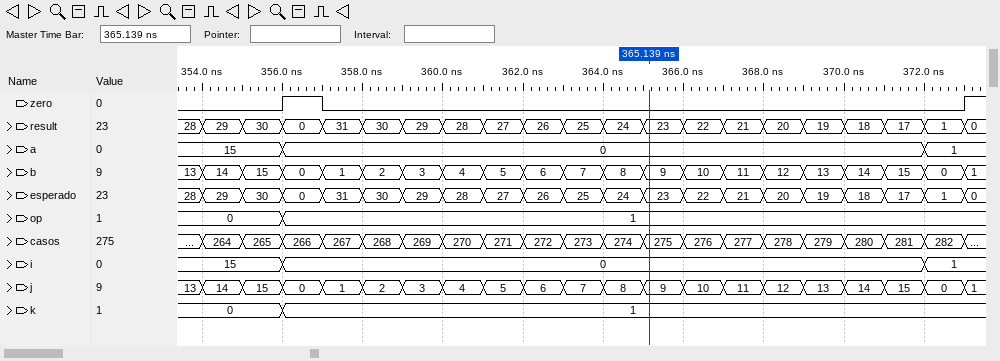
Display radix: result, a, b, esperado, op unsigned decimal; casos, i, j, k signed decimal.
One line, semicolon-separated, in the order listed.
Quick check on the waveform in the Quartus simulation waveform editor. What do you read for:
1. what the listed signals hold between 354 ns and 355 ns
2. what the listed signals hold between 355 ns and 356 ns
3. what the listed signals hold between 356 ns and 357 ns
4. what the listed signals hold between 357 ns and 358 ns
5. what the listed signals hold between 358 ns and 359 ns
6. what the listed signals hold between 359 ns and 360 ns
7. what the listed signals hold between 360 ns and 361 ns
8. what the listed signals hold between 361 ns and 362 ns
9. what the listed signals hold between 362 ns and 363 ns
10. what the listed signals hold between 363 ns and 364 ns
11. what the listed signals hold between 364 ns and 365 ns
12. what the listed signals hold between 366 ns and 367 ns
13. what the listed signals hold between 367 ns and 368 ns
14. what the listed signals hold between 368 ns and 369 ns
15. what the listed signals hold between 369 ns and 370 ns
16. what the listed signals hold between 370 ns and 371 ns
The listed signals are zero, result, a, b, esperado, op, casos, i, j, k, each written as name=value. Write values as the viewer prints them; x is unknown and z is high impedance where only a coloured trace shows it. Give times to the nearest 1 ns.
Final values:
zero=0, result=29, a=15, b=14, esperado=29, op=0, casos=264, i=15, j=14, k=0; zero=0, result=30, a=15, b=15, esperado=30, op=0, casos=265, i=15, j=15, k=0; zero=1, result=0, a=0, b=0, esperado=0, op=1, casos=266, i=0, j=0, k=1; zero=0, result=31, a=0, b=1, esperado=31, op=1, casos=267, i=0, j=1, k=1; zero=0, result=30, a=0, b=2, esperado=30, op=1, casos=268, i=0, j=2, k=1; zero=0, result=29, a=0, b=3, esperado=29, op=1, casos=269, i=0, j=3, k=1; zero=0, result=28, a=0, b=4, esperado=28, op=1, casos=270, i=0, j=4, k=1; zero=0, result=27, a=0, b=5, esperado=27, op=1, casos=271, i=0, j=5, k=1; zero=0, result=26, a=0, b=6, esperado=26, op=1, casos=272, i=0, j=6, k=1; zero=0, result=25, a=0, b=7, esperado=25, op=1, casos=273, i=0, j=7, k=1; zero=0, result=24, a=0, b=8, esperado=24, op=1, casos=274, i=0, j=8, k=1; zero=0, result=22, a=0, b=10, esperado=22, op=1, casos=276, i=0, j=10, k=1; zero=0, result=21, a=0, b=11, esperado=21, op=1, casos=277, i=0, j=11, k=1; zero=0, result=20, a=0, b=12, esperado=20, op=1, casos=278, i=0, j=12, k=1; zero=0, result=19, a=0, b=13, esperado=19, op=1, casos=279, i=0, j=13, k=1; zero=0, result=18, a=0, b=14, esperado=18, op=1, casos=280, i=0, j=14, k=1
